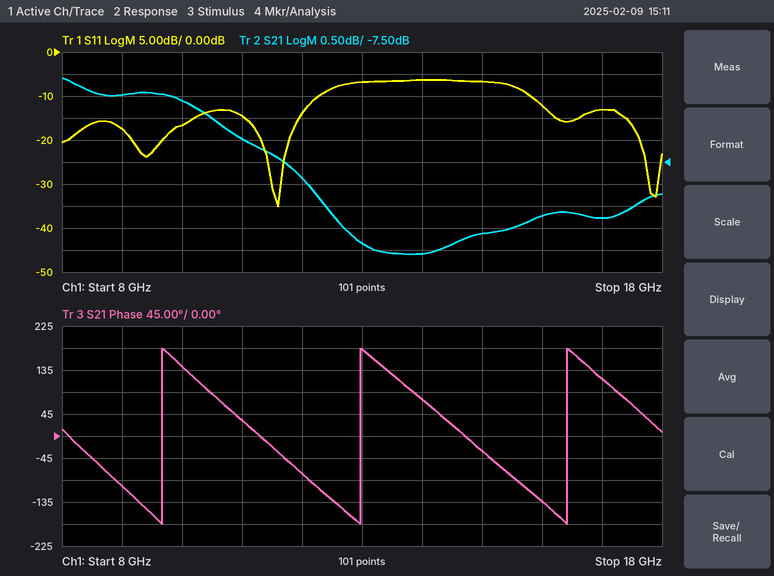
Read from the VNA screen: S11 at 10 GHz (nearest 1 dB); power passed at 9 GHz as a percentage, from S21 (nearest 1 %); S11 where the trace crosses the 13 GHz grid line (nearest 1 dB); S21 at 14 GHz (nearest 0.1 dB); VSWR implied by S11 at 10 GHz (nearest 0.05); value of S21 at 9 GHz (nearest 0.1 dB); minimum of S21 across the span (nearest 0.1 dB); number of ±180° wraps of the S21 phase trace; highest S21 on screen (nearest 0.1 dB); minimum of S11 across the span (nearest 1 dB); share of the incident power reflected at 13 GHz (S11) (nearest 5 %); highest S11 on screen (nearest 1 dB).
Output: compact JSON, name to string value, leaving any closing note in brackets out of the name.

{"S11 at 10 GHz": "-17 dB", "power passed at 9 GHz as a percentage, from S21": "25 %", "S11 where the trace crosses the 13 GHz grid line": "-7 dB", "S21 at 14 GHz": "-9.6 dB", "VSWR implied by S11 at 10 GHz": "1.35", "value of S21 at 9 GHz": "-6.0 dB", "minimum of S21 across the span": "-9.6 dB", "number of ±180° wraps of the S21 phase trace": "3", "highest S21 on screen": "-5.6 dB", "minimum of S11 across the span": "-35 dB", "share of the incident power reflected at 13 GHz (S11)": "20 %", "highest S11 on screen": "-6 dB"}
